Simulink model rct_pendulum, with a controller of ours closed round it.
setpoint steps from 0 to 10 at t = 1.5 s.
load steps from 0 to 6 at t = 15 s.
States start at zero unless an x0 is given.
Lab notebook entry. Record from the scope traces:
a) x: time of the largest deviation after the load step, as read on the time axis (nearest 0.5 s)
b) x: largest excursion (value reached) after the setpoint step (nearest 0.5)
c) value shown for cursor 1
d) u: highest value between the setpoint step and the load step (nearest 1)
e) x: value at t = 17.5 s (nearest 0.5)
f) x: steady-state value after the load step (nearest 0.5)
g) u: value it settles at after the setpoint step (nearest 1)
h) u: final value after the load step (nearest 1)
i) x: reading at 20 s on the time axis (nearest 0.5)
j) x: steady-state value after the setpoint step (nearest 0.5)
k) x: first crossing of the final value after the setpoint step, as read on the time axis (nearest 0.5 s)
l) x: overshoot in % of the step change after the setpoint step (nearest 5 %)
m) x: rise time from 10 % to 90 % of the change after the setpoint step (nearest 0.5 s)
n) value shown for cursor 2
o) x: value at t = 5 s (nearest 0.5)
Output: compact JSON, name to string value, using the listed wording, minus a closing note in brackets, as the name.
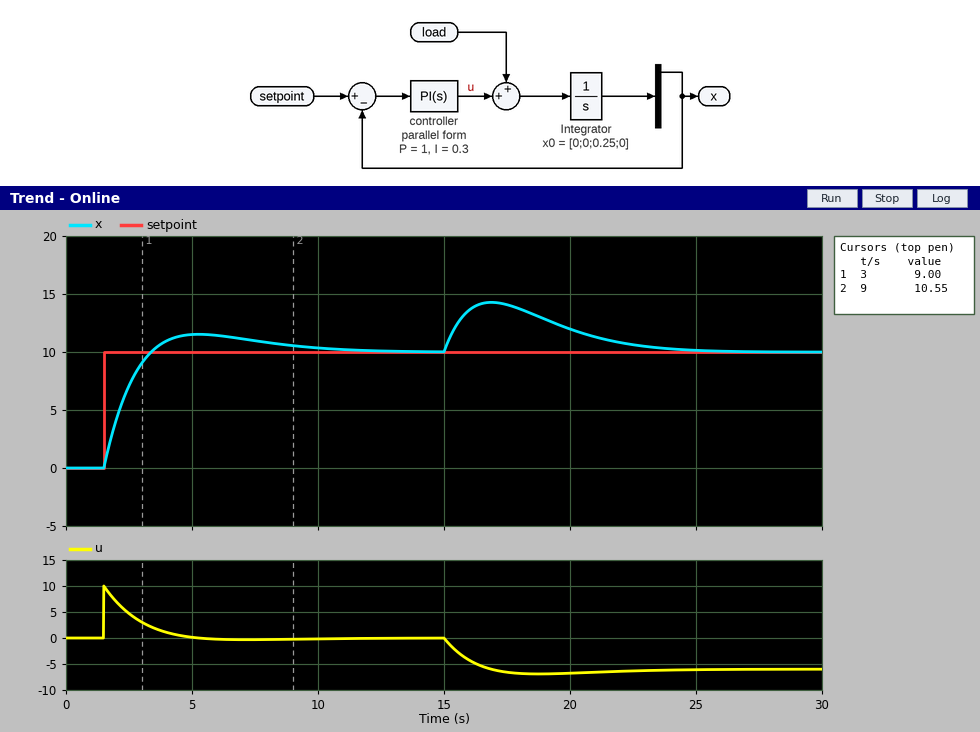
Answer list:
{"x: time of the largest deviation after the load step, as read on the time axis": "17.0 s", "x: largest excursion (value reached) after the setpoint step": "11.5", "value shown for cursor 1": "9.00", "u: highest value between the setpoint step and the load step": "10", "x: value at t = 17.5 s": "14.0", "x: steady-state value after the load step": "10.0", "u: value it settles at after the setpoint step": "0", "u: final value after the load step": "-6", "x: reading at 20 s on the time axis": "12.0", "x: steady-state value after the setpoint step": "10.0", "x: first crossing of the final value after the setpoint step, as read on the time axis": "3.5 s", "x: overshoot in % of the step change after the setpoint step": "15 %", "x: rise time from 10 % to 90 % of the change after the setpoint step": "1.5 s", "value shown for cursor 2": "10.55", "x: value at t = 5 s": "11.5"}
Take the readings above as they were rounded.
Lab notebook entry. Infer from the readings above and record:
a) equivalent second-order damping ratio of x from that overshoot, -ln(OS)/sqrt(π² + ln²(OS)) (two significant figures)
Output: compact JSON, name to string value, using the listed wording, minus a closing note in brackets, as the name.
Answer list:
{"equivalent second-order damping ratio of x from that overshoot, -ln(OS)/sqrt(π² + ln²(OS))": "0.52"}
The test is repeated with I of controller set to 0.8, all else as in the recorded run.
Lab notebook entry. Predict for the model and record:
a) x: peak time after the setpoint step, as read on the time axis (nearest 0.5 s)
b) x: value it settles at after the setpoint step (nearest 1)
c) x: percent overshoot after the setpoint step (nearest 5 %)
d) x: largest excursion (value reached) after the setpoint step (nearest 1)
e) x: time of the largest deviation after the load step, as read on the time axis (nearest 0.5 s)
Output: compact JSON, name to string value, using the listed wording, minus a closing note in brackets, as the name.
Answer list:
{"x: peak time after the setpoint step, as read on the time axis": "4.0 s", "x: value it settles at after the setpoint step": "10", "x: percent overshoot after the setpoint step": "25 %", "x: largest excursion (value reached) after the setpoint step": "13", "x: time of the largest deviation after the load step, as read on the time axis": "16.5 s"}
